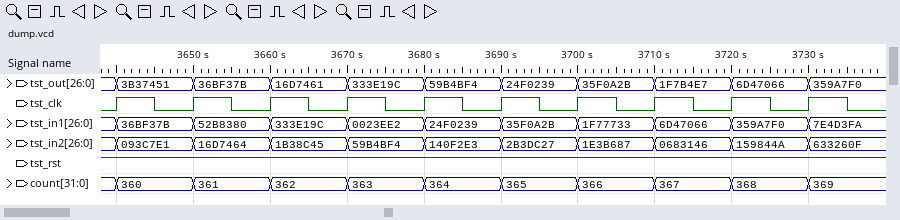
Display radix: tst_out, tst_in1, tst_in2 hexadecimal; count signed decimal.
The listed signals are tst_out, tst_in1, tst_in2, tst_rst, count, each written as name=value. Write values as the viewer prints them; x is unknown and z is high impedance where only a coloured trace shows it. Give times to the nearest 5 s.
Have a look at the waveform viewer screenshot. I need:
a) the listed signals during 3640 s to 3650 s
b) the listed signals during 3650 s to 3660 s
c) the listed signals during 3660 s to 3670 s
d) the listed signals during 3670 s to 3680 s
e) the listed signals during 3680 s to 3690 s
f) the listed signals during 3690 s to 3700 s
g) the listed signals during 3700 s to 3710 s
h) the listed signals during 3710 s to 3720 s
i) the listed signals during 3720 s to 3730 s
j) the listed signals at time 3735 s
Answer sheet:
tst_out=3B37451, tst_in1=36BF37B, tst_in2=093C7E1, tst_rst=1, count=360
tst_out=36BF37B, tst_in1=52B8380, tst_in2=16D7464, tst_rst=1, count=361
tst_out=16D7461, tst_in1=333E19C, tst_in2=1B38C45, tst_rst=1, count=362
tst_out=333E19C, tst_in1=0023EE2, tst_in2=59B4BF4, tst_rst=1, count=363
tst_out=59B4BF4, tst_in1=24F0239, tst_in2=140F2E3, tst_rst=1, count=364
tst_out=24F0239, tst_in1=35F0A2B, tst_in2=2B3DC27, tst_rst=1, count=365
tst_out=35F0A2B, tst_in1=1F77733, tst_in2=1E3B687, tst_rst=1, count=366
tst_out=1F7B4E7, tst_in1=6D47066, tst_in2=0683146, tst_rst=1, count=367
tst_out=6D47066, tst_in1=359A7F0, tst_in2=159844A, tst_rst=1, count=368
tst_out=359A7F0, tst_in1=7E4D3FA, tst_in2=633260F, tst_rst=1, count=369
